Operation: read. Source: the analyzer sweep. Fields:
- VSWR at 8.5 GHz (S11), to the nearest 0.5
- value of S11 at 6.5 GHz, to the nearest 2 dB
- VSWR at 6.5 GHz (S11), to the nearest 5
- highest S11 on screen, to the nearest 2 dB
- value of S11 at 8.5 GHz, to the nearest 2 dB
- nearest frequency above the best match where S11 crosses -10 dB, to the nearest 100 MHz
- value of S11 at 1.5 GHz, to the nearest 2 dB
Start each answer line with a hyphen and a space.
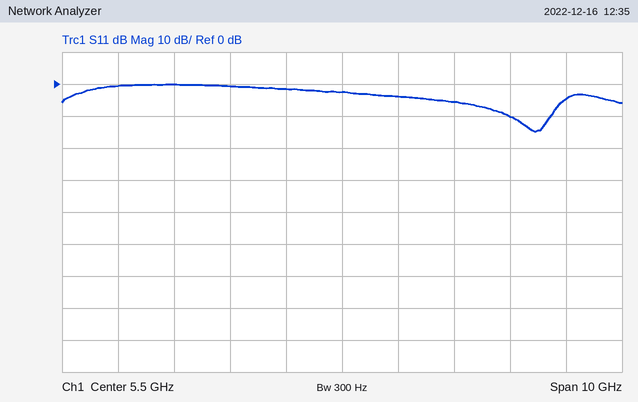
- 2.0
- -4 dB
- 5
- 0 dB
- -10 dB
- 9.2 GHz
- 0 dB
